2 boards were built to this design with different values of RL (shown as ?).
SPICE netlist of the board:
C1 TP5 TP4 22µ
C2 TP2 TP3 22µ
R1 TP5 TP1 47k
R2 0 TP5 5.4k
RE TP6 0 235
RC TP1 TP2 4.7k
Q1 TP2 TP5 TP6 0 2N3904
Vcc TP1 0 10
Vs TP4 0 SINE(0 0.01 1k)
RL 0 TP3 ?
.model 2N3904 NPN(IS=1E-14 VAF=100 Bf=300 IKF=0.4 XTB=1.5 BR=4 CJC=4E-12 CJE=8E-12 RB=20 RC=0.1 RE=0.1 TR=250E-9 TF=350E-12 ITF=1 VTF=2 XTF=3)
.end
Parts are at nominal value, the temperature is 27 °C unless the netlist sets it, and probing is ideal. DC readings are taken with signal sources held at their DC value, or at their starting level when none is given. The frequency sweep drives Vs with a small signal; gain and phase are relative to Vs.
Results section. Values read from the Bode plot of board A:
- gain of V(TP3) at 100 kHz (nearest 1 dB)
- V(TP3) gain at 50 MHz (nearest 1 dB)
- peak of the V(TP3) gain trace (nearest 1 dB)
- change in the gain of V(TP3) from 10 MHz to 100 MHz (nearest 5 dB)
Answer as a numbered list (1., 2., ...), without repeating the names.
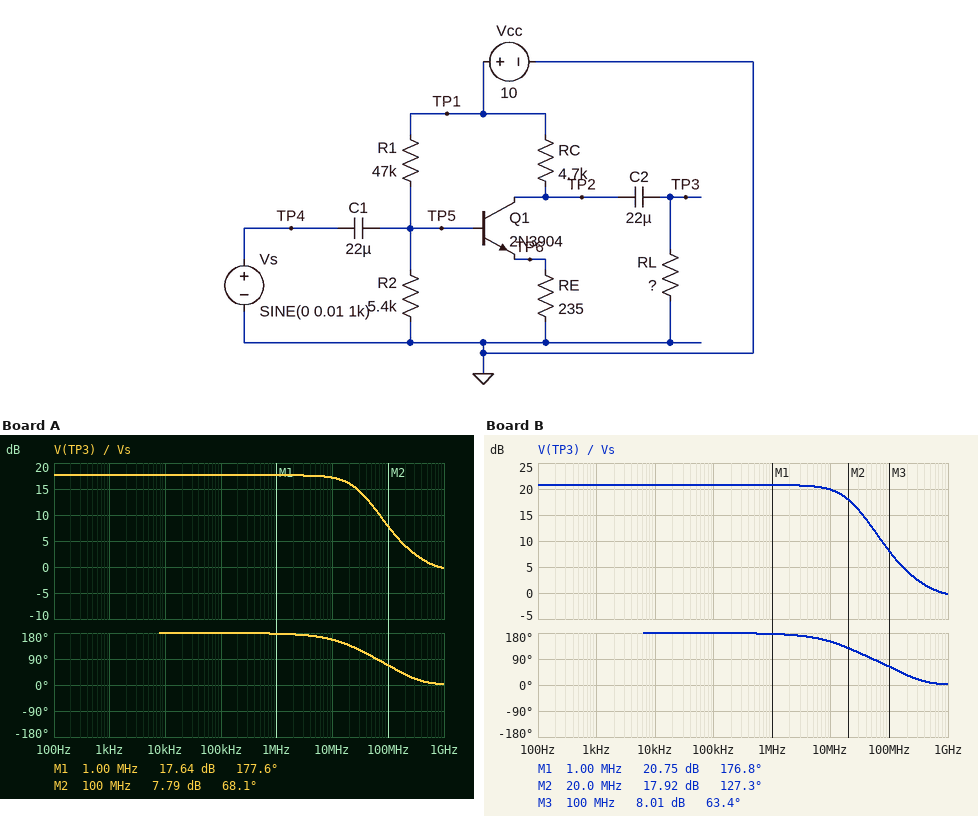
1. 18 dB
2. 12 dB
3. 18 dB
4. -10 dB
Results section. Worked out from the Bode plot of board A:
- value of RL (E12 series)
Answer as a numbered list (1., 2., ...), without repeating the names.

1. 3.3 kΩ
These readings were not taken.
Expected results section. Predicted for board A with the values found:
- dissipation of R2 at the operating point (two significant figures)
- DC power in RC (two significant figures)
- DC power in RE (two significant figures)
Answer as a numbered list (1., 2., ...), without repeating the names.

1. 190 µW
2. 9.9 mW
3. 500 µW
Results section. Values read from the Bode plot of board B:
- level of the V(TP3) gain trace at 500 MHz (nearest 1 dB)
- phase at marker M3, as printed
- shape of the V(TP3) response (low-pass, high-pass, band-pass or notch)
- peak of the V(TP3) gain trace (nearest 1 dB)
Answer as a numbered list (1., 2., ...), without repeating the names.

1. 1 dB
2. 63.4 deg
3. low-pass
4. 21 dB
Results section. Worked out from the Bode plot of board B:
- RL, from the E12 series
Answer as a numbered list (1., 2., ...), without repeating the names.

1. 6.8 kΩ
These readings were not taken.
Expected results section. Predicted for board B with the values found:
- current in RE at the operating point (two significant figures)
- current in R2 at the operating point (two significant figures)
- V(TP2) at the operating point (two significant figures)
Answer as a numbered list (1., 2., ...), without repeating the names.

1. 1.5 mA
2. 190 µA
3. 3.2 V
